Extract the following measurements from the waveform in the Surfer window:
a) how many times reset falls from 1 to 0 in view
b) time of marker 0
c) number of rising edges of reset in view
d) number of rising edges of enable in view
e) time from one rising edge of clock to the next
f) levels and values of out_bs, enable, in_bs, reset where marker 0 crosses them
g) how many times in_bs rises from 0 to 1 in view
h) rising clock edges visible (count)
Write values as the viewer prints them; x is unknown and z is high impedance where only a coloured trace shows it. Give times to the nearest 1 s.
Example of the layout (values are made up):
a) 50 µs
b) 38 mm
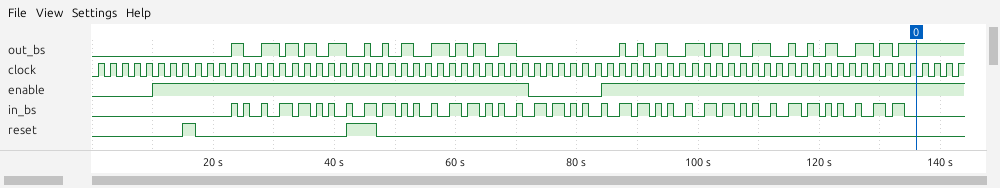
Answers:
a) 2
b) 136 s
c) 2
d) 2
e) 2 s
f) out_bs=1, enable=1, in_bs=0, reset=0
g) 40
h) 72
